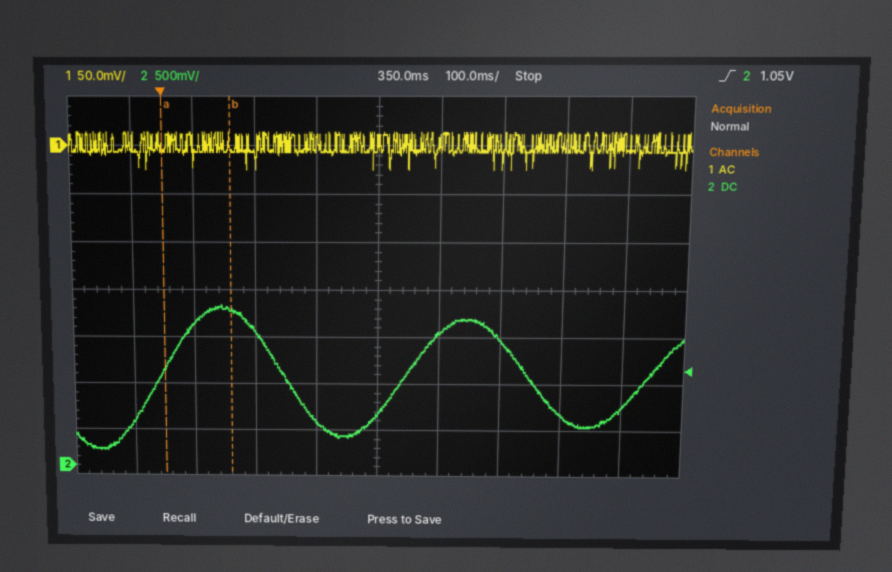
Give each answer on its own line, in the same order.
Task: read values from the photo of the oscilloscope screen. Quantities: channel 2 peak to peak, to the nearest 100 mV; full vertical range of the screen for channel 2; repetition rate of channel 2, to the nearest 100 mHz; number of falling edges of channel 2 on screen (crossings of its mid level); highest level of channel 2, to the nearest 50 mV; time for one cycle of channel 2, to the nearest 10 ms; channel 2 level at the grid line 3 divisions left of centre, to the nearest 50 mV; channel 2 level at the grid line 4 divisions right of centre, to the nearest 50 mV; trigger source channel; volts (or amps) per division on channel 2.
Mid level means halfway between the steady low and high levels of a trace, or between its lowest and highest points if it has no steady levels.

1.60 V
4 V
2.5 Hz
2
1.75 V
400 ms
1.55 V
650 mV
channel 2
500 mV
